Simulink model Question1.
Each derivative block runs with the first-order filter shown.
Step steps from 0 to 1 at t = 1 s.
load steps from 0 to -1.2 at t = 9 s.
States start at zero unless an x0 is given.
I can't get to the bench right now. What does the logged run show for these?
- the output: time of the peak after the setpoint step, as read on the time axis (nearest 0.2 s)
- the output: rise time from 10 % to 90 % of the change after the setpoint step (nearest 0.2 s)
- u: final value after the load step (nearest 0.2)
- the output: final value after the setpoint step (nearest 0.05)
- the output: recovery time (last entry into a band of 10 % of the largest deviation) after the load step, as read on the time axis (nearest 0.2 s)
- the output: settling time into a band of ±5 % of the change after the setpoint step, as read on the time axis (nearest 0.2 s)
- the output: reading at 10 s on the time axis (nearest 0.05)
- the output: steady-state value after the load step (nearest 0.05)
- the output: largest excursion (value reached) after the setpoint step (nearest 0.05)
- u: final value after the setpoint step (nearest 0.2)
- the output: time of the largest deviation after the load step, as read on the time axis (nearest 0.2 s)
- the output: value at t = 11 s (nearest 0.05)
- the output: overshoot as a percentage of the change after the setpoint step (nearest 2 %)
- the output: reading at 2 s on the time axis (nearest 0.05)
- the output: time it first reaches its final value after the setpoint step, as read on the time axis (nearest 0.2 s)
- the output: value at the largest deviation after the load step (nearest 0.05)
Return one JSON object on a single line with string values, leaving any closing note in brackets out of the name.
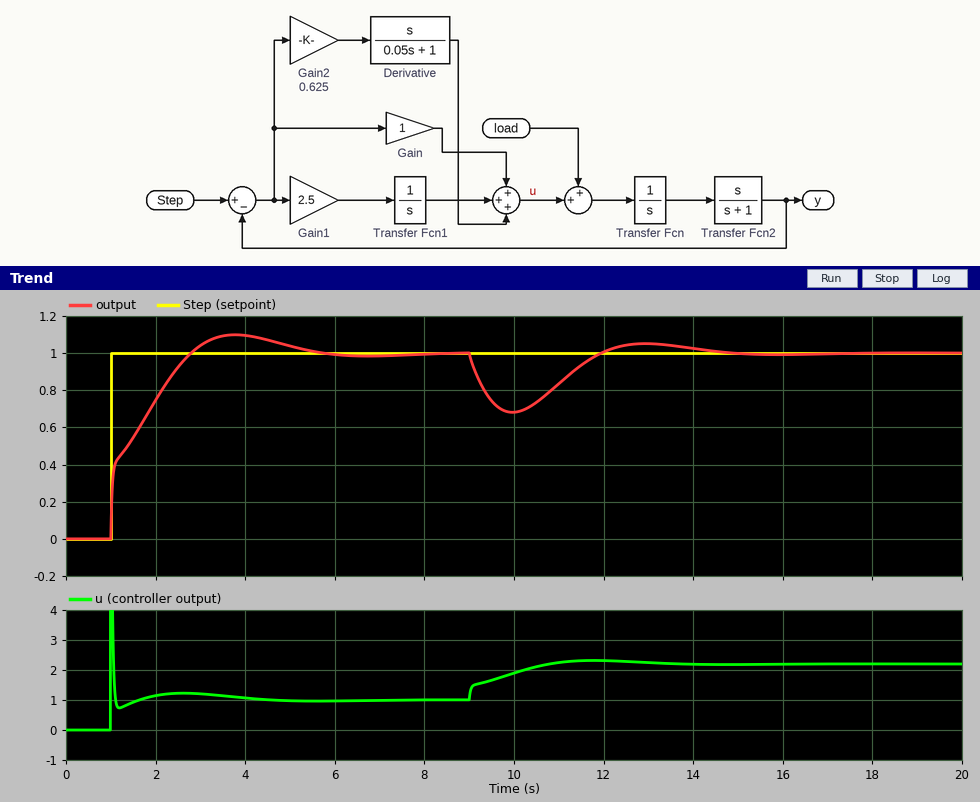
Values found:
{"the output: time of the peak after the setpoint step, as read on the time axis": "3.8 s", "the output: rise time from 10 % to 90 % of the change after the setpoint step": "1.4 s", "u: final value after the load step": "2.2", "the output: final value after the setpoint step": "1.00", "the output: recovery time (last entry into a band of 10 % of the largest deviation) after the load step, as read on the time axis": "13.8 s", "the output: settling time into a band of ±5 % of the change after the setpoint step, as read on the time axis": "4.8 s", "the output: reading at 10 s on the time axis": "0.70", "the output: steady-state value after the load step": "1.00", "the output: largest excursion (value reached) after the setpoint step": "1.10", "u: final value after the setpoint step": "1.0", "the output: time of the largest deviation after the load step, as read on the time axis": "10.0 s", "the output: value at t = 11 s": "0.85", "the output: overshoot as a percentage of the change after the setpoint step": "10 %", "the output: reading at 2 s on the time axis": "0.75", "the output: time it first reaches its final value after the setpoint step, as read on the time axis": "2.8 s", "the output: value at the largest deviation after the load step": "0.70"}
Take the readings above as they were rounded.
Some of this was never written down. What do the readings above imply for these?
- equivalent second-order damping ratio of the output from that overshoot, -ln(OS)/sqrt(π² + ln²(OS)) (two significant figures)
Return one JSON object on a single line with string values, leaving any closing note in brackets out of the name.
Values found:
{"equivalent second-order damping ratio of the output from that overshoot, -ln(OS)/sqrt(π² + ln²(OS))": "0.59"}
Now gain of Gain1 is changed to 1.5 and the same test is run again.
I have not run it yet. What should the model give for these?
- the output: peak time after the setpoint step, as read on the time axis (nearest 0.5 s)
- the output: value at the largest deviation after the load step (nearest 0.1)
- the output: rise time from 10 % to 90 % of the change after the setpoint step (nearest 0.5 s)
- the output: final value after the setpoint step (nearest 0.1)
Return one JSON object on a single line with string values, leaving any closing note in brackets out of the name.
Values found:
{"the output: peak time after the setpoint step, as read on the time axis": "5.0 s", "the output: value at the largest deviation after the load step": "0.6", "the output: rise time from 10 % to 90 % of the change after the setpoint step": "2.0 s", "the output: final value after the setpoint step": "1.0"}
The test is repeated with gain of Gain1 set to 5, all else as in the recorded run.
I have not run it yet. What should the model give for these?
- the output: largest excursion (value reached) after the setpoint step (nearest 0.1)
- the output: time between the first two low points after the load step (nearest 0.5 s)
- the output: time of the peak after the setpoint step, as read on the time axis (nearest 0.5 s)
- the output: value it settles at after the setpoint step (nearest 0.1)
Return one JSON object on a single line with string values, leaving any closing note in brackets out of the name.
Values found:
{"the output: largest excursion (value reached) after the setpoint step": "1.2", "the output: time between the first two low points after the load step": "4.0 s", "the output: time of the peak after the setpoint step, as read on the time axis": "3.0 s", "the output: value it settles at after the setpoint step": "1.0"}
